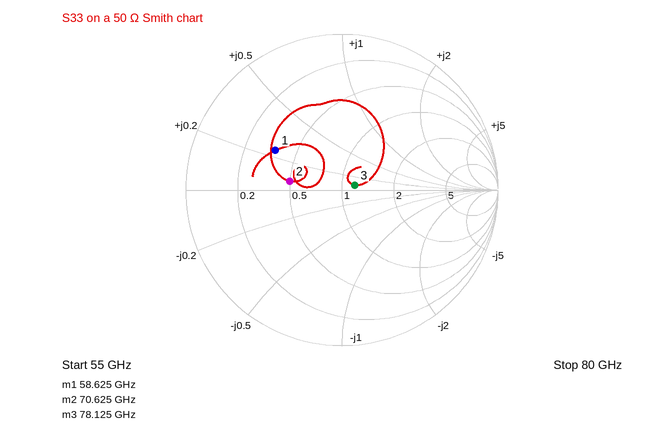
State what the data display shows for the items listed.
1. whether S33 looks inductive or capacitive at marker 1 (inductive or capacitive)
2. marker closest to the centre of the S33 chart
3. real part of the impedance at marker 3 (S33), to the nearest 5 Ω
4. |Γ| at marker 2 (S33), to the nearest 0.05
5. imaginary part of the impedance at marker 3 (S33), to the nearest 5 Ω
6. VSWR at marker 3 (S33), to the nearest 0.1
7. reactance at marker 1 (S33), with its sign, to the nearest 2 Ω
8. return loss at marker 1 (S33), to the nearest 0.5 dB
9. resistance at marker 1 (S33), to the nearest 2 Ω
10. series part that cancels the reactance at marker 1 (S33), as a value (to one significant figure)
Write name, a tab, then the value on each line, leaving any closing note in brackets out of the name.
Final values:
whether S33 looks inductive or capacitive at marker 1	inductive
marker closest to the centre of the S33 chart	marker 3
real part of the impedance at marker 3 (S33), to the nearest 5 Ω	60 Ω
|Γ| at marker 2 (S33), to the nearest 0.05	0.35
imaginary part of the impedance at marker 3 (S33), to the nearest 5 Ω	+5 Ω
VSWR at marker 3 (S33), to the nearest 0.1	1.2
reactance at marker 1 (S33), with its sign, to the nearest 2 Ω	+12 Ω
return loss at marker 1 (S33), to the nearest 0.5 dB	6.0 dB
resistance at marker 1 (S33), to the nearest 2 Ω	18 Ω
series part that cancels the reactance at marker 1 (S33), as a value	200 fF
